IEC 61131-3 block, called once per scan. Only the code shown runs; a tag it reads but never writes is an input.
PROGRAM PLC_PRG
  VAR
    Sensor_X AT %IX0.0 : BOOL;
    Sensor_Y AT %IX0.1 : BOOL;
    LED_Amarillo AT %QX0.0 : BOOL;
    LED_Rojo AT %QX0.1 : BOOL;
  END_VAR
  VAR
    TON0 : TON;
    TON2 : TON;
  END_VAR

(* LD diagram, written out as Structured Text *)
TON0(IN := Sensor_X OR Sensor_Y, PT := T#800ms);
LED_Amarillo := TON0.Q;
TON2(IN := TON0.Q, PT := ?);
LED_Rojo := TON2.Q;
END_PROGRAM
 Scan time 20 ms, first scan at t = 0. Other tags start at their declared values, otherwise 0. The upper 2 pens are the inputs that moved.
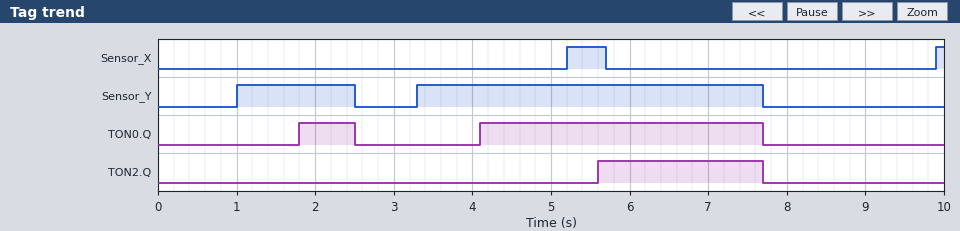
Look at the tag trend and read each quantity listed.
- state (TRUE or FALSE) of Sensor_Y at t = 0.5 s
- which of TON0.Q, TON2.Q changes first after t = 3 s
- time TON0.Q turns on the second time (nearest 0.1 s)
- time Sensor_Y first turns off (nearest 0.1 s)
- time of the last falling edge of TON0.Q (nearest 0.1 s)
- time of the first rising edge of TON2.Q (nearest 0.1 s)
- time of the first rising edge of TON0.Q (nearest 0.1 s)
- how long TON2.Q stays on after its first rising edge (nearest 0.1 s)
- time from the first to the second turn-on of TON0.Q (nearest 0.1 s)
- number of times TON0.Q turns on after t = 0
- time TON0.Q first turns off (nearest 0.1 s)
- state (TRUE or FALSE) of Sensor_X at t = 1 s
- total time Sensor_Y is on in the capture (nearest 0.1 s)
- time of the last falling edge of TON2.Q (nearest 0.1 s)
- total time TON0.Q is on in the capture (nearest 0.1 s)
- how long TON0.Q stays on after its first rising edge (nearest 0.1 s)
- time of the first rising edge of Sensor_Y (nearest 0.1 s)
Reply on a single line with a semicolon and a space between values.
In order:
FALSE; TON0.Q; 4.1 s; 2.5 s; 7.7 s; 5.6 s; 1.8 s; 2.1 s; 2.3 s; 2; 2.5 s; FALSE; 5.9 s; 7.7 s; 4.3 s; 0.7 s; 1.0 s
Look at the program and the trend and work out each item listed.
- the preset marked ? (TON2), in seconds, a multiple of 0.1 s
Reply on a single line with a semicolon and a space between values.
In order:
1.5 s
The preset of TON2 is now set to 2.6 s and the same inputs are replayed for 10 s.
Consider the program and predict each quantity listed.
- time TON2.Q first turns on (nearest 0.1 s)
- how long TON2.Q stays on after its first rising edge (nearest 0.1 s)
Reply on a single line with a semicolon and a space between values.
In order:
6.7 s; 1.0 s
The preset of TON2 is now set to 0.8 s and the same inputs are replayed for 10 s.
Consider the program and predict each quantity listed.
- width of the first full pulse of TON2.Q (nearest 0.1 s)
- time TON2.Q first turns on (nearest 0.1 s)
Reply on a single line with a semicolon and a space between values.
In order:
2.8 s; 4.9 s
